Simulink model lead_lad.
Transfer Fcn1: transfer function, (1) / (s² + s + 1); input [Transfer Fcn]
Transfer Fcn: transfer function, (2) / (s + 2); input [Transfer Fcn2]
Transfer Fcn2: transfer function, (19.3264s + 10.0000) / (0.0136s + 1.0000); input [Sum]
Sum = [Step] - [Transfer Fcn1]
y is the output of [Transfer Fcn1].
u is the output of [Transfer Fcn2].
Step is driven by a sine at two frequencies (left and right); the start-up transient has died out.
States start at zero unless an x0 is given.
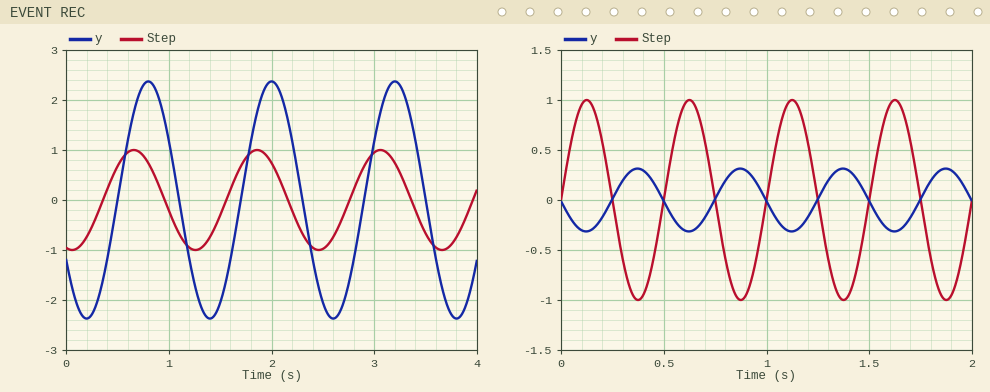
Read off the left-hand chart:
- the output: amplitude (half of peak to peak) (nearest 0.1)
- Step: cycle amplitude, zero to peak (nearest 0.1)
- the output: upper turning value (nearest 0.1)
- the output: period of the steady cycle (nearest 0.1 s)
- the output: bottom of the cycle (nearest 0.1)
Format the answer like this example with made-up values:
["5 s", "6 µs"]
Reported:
["2.4", "1.0", "2.4", "1.2 s", "-2.4"]
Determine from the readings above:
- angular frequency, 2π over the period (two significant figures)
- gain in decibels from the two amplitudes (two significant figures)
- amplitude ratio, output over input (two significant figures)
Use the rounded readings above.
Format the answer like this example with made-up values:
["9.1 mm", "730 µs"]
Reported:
["5.2 rad/s", "7.6 dB", "2.4"]
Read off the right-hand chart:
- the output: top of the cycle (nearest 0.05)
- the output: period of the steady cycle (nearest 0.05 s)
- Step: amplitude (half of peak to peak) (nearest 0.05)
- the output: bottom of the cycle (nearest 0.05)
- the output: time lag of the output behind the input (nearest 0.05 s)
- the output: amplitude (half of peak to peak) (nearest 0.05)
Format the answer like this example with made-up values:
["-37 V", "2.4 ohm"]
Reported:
["0.30", "0.50 s", "1.00", "-0.30", "0.25 s", "0.30"]
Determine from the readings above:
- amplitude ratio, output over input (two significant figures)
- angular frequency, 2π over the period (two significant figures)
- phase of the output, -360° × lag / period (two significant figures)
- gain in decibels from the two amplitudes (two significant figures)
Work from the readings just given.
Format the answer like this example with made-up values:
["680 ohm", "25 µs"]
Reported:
["0.30", "13 rad/s", "-180°", "-10 dB"]
